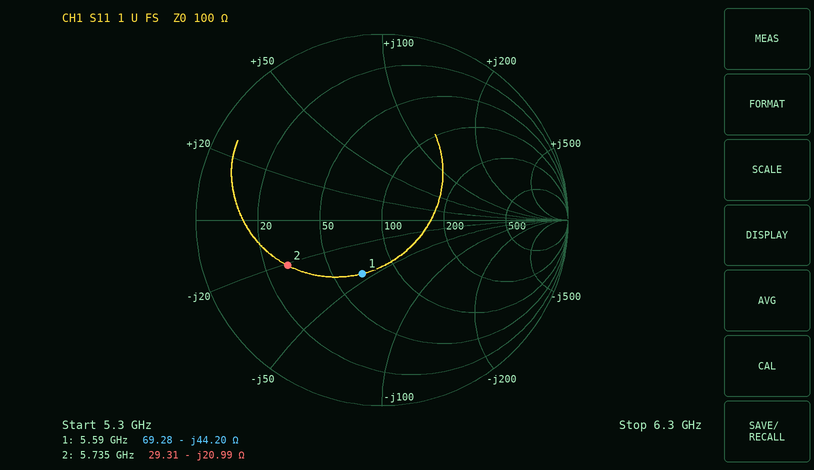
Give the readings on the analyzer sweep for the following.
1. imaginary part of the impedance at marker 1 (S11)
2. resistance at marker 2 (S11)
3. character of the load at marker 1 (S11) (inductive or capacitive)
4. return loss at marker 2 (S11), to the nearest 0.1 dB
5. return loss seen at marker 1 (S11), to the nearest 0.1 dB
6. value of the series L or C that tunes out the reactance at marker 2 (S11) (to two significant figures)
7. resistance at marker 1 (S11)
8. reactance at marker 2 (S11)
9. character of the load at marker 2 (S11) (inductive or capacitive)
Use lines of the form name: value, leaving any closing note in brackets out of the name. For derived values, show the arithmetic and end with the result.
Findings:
imaginary part of the impedance at marker 1: -44.20 Ω
resistance at marker 2: 29.31 Ω
character of the load at marker 1 (S11): capacitive
return loss at marker 2 (S11), to the nearest 0.1 dB: 5.0 dB
return loss seen at marker 1 (S11), to the nearest 0.1 dB: 10.2 dB
value of the series L or C that tunes out the reactance at marker 2 (S11): L = 20.99 Ω/(2π × 5.735 GHz) ≈ 583 pH, so 580 pH to two significant figures
resistance at marker 1: 69.28 Ω
reactance at marker 2: -20.99 Ω
character of the load at marker 2 (S11): capacitive
